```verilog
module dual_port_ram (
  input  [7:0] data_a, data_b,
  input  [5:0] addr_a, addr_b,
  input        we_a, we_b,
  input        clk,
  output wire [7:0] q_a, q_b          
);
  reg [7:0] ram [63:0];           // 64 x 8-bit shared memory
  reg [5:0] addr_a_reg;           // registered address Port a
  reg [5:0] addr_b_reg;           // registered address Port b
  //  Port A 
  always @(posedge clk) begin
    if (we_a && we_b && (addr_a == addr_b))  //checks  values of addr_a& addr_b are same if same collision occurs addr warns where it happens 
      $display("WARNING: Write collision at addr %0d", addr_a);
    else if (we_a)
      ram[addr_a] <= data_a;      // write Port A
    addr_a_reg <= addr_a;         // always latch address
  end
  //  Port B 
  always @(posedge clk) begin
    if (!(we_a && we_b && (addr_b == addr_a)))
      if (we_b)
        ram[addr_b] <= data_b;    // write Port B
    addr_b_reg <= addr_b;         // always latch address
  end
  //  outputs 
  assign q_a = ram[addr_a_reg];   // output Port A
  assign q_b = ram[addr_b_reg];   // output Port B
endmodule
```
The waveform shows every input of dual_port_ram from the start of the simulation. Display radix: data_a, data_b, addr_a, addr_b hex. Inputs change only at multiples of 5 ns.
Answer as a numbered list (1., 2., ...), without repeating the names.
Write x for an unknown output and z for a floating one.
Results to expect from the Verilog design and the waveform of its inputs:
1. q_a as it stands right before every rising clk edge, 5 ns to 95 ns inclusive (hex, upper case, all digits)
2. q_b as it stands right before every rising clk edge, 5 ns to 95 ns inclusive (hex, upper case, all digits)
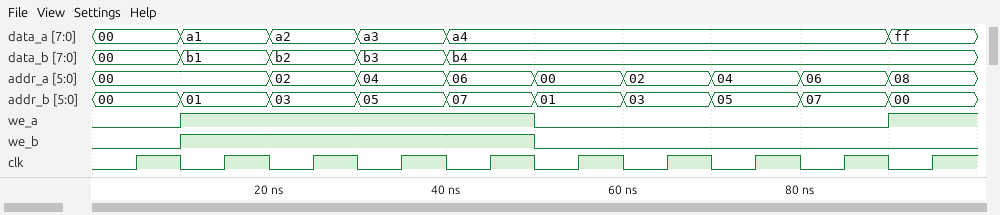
1. x, x, A1, A2, A3, A4, A1, A2, A3, A4
2. x, x, B1, B2, B3, B4, B1, B2, B3, B4
